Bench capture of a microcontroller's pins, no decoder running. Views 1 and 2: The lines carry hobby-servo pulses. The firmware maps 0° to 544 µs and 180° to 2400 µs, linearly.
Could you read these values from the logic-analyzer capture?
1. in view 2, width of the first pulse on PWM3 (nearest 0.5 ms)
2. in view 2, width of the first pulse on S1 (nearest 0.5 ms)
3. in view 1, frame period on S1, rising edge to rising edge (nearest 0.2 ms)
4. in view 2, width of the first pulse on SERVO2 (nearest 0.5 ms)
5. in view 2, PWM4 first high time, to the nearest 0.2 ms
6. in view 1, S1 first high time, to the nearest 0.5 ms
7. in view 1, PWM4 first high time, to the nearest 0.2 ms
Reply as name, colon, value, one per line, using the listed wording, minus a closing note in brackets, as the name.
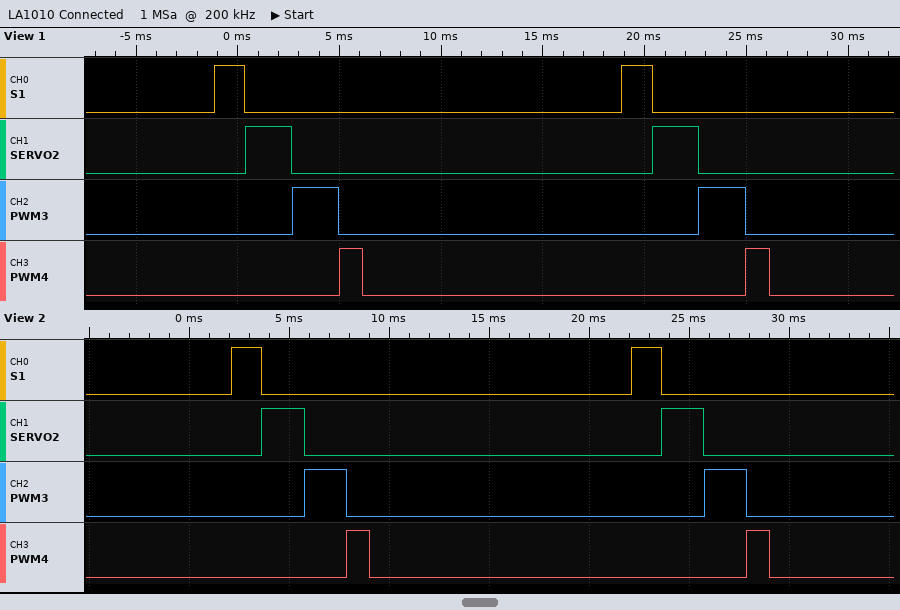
in view 2, width of the first pulse on PWM3: 2.0 ms
in view 2, width of the first pulse on S1: 1.5 ms
in view 1, frame period on S1, rising edge to rising edge: 20.0 ms
in view 2, width of the first pulse on SERVO2: 2.0 ms
in view 2, PWM4 first high time, to the nearest 0.2 ms: 1.2 ms
in view 1, S1 first high time, to the nearest 0.5 ms: 1.5 ms
in view 1, PWM4 first high time, to the nearest 0.2 ms: 1.2 ms
